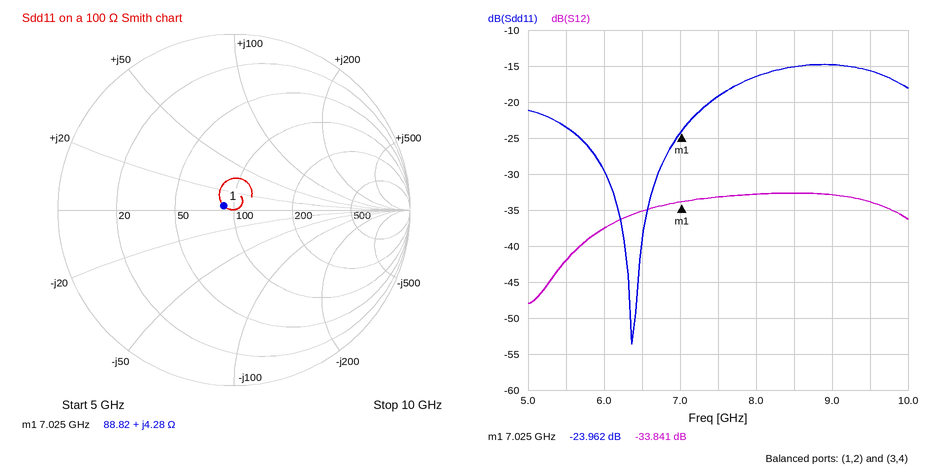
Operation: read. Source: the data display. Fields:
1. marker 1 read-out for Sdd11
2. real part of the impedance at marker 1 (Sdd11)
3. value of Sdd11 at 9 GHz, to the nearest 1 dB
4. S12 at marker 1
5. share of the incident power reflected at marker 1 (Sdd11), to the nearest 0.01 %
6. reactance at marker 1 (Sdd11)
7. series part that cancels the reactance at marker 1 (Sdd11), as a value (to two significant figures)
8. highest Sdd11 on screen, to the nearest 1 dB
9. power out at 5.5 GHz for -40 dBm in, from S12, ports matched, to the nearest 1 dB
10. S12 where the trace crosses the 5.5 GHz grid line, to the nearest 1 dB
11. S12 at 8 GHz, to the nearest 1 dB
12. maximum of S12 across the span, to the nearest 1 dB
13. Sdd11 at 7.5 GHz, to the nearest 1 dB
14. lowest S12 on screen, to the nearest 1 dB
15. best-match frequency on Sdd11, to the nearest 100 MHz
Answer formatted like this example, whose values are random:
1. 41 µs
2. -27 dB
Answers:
1. -23.962 dB
2. 88.82 Ω
3. -15 dB
4. -33.841 dB
5. 0.40 %
6. +4.28 Ω
7. 5.3 pF
8. -15 dB
9. -82 dBm
10. -42 dB
11. -33 dB
12. -33 dB
13. -19 dB
14. -48 dB
15. 6.4 GHz
